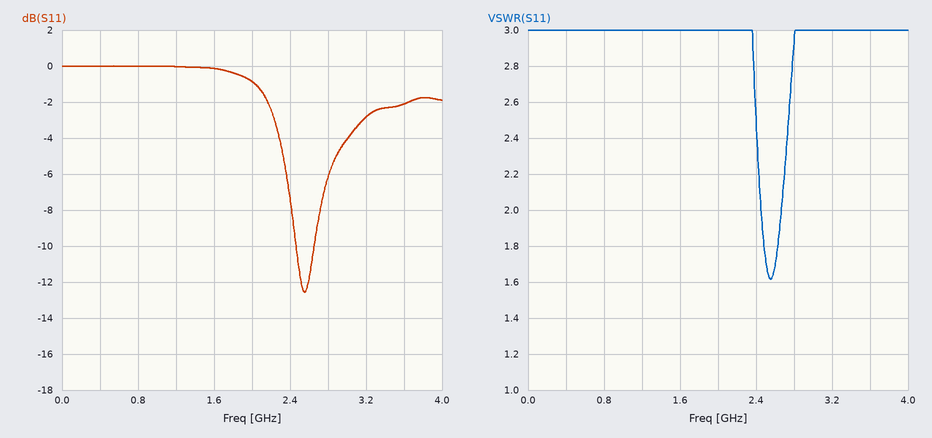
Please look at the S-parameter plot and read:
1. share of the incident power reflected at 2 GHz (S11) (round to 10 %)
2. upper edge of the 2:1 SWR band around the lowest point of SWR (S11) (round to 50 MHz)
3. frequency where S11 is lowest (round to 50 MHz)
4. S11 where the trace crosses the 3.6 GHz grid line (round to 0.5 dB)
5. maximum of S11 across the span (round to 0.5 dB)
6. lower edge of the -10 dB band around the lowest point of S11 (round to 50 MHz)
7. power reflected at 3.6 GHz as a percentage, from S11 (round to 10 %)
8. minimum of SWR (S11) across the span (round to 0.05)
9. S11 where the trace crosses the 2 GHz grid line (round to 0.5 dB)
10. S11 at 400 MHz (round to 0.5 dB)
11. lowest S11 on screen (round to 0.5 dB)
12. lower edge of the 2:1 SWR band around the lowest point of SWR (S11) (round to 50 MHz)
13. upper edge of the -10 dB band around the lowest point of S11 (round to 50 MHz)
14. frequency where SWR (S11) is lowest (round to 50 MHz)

80 %
2.65 GHz
2.55 GHz
-2.0 dB
0.0 dB
2.45 GHz
60 %
1.60
-1.0 dB
0.0 dB
-12.5 dB
2.45 GHz
2.65 GHz
2.55 GHz
